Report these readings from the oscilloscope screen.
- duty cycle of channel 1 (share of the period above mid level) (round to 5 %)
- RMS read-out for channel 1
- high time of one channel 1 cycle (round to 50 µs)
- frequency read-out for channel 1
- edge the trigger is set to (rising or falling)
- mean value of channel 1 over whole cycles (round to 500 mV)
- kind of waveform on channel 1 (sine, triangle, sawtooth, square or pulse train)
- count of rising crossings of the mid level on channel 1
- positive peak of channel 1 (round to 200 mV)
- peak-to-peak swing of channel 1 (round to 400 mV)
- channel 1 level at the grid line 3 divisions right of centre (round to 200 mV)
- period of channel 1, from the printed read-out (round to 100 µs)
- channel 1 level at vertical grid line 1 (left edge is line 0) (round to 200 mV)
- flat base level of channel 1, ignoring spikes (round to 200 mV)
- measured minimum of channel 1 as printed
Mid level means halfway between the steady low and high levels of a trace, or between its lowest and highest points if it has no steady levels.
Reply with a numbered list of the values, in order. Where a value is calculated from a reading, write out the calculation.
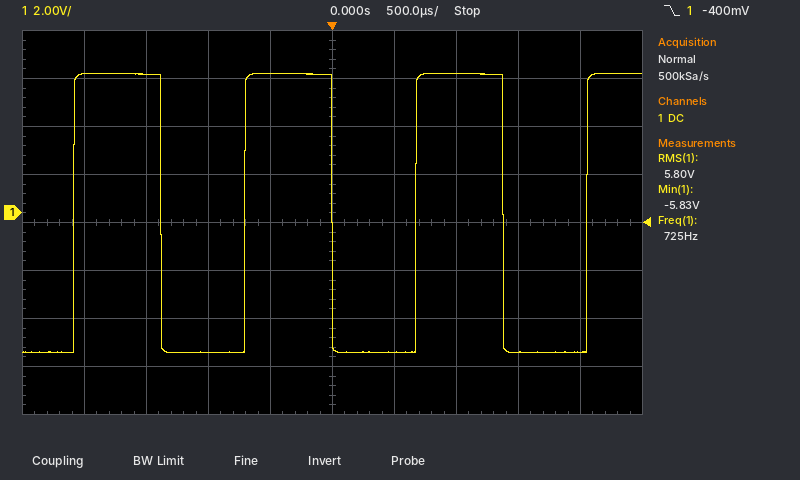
1. 50 %
2. 5.80 V
3. 700 µs
4. 725 Hz
5. falling
6. -5.8 V + 0.5 × (5.8 V − (-5.8 V)) ≈ 0.0 V
7. square
8. 4
9. 5.8 V
10. 11.6 V
11. -5.8 V
12. 1 / 725 Hz ≈ 1.4 ms
13. 5.8 V
14. -5.8 V
15. -5.83 V
